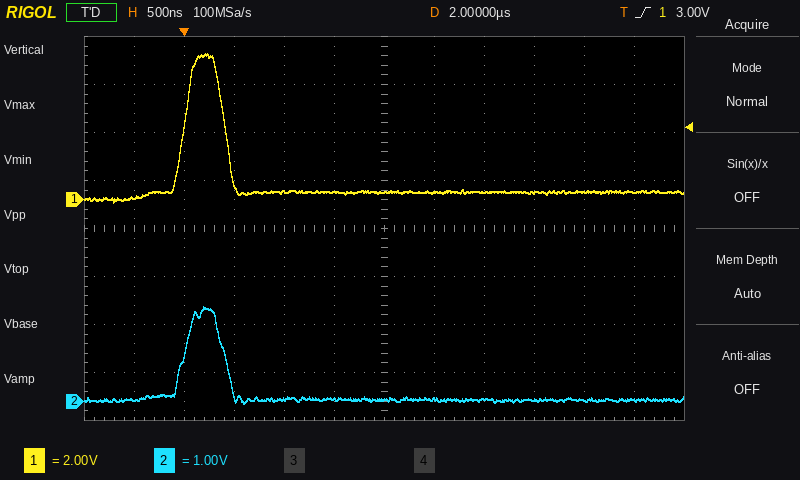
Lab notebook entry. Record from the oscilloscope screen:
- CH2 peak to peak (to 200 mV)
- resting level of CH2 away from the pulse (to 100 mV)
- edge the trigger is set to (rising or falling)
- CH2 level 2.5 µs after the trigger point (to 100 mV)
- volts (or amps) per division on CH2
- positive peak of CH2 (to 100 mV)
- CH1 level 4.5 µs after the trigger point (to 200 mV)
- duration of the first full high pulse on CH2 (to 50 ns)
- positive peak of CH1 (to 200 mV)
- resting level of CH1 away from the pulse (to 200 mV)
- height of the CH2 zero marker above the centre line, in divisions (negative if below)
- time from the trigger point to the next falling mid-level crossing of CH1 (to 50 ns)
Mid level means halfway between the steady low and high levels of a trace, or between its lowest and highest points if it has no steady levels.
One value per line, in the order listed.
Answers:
2.0 V
0.0 V
rising
0.0 V
1 V
2.0 V
400 mV
400 ns
6.0 V
400 mV
-3.6 div
400 ns
